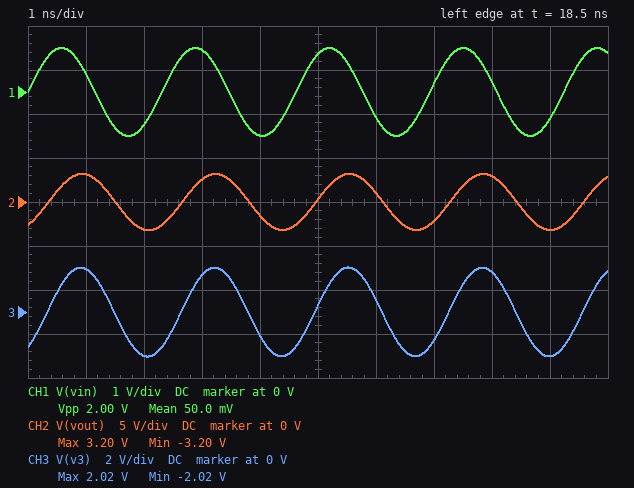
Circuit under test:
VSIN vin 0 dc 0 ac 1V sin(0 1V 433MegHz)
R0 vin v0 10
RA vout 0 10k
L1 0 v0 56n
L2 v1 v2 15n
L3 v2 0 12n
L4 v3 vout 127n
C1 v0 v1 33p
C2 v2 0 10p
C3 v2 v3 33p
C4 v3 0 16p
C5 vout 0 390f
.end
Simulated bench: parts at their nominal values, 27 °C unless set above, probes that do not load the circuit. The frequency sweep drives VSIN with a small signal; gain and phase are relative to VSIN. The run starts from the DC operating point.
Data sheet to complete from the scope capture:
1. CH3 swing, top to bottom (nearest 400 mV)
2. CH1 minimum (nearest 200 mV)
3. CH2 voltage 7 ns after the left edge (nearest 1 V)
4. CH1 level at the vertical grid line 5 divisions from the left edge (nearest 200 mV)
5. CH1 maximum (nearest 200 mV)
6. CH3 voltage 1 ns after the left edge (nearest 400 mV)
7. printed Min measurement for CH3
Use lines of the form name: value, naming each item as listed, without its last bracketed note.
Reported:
CH3 swing, top to bottom: 4.0 V
CH1 minimum: -1.0 V
CH2 voltage 7 ns after the left edge: -2 V
CH1 level at the vertical grid line 5 divisions from the left edge: 800 mV
CH1 maximum: 1.0 V
CH3 voltage 1 ns after the left edge: 2.0 V
printed Min measurement for CH3: -2.02 V
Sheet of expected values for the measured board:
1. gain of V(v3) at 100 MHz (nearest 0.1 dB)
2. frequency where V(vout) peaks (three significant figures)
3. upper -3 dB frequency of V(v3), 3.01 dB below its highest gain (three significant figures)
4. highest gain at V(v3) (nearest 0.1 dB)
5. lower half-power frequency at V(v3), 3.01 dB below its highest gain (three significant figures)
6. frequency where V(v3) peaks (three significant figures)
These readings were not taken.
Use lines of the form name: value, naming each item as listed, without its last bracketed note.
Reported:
gain of V(v3) at 100 MHz: -14.7 dB
frequency where V(vout) peaks: 449 MHz
upper -3 dB frequency of V(v3), 3.01 dB below its highest gain: 476 MHz
highest gain at V(v3): 6.8 dB
lower half-power frequency at V(v3), 3.01 dB below its highest gain: 414 MHz
frequency where V(v3) peaks: 447 MHz
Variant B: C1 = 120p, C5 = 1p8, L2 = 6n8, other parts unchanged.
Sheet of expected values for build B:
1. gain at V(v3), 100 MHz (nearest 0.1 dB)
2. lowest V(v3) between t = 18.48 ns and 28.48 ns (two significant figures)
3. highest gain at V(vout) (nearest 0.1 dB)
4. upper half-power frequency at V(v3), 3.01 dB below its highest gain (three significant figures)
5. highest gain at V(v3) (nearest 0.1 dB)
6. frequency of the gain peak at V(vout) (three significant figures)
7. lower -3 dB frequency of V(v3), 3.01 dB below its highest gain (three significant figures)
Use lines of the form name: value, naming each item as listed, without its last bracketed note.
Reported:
gain at V(v3), 100 MHz: -5.2 dB
lowest V(v3) between t = 18.48 ns and 28.48 ns: -1.1 V
highest gain at V(vout): 23.9 dB
upper half-power frequency at V(v3), 3.01 dB below its highest gain: 598 MHz
highest gain at V(v3): 3.9 dB
frequency of the gain peak at V(vout): 336 MHz
lower -3 dB frequency of V(v3), 3.01 dB below its highest gain: 444 MHz
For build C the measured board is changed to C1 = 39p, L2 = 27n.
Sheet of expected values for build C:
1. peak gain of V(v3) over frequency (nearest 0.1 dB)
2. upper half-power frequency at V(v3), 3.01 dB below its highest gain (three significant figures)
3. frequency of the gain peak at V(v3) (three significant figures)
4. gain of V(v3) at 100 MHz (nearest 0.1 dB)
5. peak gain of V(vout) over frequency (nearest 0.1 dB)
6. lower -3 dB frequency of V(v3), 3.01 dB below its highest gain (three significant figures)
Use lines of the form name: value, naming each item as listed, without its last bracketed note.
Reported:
peak gain of V(v3) over frequency: 11.4 dB
upper half-power frequency at V(v3), 3.01 dB below its highest gain: 400 MHz
frequency of the gain peak at V(v3): 389 MHz
gain of V(v3) at 100 MHz: -9.4 dB
peak gain of V(vout) over frequency: 14.4 dB
lower -3 dB frequency of V(v3), 3.01 dB below its highest gain: 378 MHz
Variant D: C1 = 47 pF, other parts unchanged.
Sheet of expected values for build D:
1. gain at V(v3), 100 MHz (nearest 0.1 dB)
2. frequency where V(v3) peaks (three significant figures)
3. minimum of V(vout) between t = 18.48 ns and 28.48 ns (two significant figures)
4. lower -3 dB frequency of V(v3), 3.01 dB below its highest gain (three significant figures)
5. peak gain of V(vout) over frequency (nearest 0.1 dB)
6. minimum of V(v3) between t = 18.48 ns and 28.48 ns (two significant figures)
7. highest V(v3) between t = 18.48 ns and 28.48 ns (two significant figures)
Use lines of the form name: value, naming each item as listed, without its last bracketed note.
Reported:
gain at V(v3), 100 MHz: -9.6 dB
frequency where V(v3) peaks: 438 MHz
minimum of V(vout) between t = 18.48 ns and 28.48 ns: -3.6 V
lower -3 dB frequency of V(v3), 3.01 dB below its highest gain: 408 MHz
peak gain of V(vout) over frequency: 11.4 dB
minimum of V(v3) between t = 18.48 ns and 28.48 ns: -2.3 V
highest V(v3) between t = 18.48 ns and 28.48 ns: 2.3 V
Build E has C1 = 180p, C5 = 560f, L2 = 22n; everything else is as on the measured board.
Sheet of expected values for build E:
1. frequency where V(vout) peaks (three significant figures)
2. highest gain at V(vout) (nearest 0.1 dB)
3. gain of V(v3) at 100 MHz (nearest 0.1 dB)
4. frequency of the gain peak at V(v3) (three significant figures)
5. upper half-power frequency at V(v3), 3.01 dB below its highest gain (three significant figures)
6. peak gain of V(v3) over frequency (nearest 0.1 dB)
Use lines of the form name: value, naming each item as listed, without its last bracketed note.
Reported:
frequency where V(vout) peaks: 393 MHz
highest gain at V(vout): 15.6 dB
gain of V(v3) at 100 MHz: -10.7 dB
frequency of the gain peak at V(v3): 392 MHz
upper half-power frequency at V(v3), 3.01 dB below its highest gain: 405 MHz
peak gain of V(v3) over frequency: 10.7 dB
